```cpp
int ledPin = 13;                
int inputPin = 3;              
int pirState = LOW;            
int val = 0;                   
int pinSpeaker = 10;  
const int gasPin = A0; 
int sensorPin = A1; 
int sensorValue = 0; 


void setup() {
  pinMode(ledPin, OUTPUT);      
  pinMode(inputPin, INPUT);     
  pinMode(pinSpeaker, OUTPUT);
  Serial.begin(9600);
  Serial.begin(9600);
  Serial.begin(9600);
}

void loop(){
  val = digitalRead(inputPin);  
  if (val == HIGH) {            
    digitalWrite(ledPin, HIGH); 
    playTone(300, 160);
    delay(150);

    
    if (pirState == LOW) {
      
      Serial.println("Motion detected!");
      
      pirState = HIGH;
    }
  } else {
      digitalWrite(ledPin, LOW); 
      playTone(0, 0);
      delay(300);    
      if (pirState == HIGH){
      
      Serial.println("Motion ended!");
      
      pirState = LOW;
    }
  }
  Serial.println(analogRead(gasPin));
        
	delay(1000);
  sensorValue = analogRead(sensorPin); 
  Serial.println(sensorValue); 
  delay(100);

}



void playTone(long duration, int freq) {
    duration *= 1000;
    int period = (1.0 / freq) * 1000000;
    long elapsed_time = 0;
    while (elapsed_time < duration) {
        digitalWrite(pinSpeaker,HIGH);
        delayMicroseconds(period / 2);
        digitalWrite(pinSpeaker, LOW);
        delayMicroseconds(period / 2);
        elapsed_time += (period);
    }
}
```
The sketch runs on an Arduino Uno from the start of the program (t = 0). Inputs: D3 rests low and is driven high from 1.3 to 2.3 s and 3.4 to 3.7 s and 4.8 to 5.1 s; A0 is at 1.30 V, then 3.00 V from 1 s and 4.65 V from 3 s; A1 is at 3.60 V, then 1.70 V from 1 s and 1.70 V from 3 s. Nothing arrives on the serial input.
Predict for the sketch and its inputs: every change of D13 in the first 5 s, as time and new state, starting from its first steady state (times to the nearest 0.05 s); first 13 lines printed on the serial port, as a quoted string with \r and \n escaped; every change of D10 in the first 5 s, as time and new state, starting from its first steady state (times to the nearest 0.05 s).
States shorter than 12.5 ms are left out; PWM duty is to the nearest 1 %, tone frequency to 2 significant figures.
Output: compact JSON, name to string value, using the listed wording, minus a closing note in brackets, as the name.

{"every change of D13 in the first 5 s, as time and new state, starting from its first steady state": "0 s low; 1.4 s high; 2.95 s low", "first 13 lines printed on the serial port, as a quoted string with \\r and \\n escaped": "\"266\\r\\n348\\r\\nMotion detected!\\r\\n614\\r\\n348\\r\\nMotion ended!\\r\\n952\\r\\n348\\r\\n952\\r\\n348\\r\\n952\\r\\n348\\r\\n952\\r\\n\"", "every change of D10 in the first 5 s, as time and new state, starting from its first steady state": "0 s low; 1.4 s tone 160 Hz; 1.7 s low"}
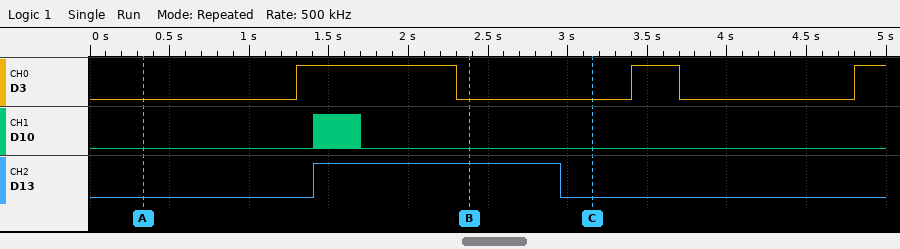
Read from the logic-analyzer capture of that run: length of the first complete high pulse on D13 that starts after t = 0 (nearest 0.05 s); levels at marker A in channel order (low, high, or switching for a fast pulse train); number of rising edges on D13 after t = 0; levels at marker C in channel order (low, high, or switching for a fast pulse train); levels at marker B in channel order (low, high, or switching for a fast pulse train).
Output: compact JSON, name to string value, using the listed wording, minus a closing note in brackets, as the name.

{"length of the first complete high pulse on D13 that starts after t = 0": "1.55 s", "levels at marker A in channel order": "D3 low, D10 low, D13 low", "number of rising edges on D13 after t = 0": "1", "levels at marker C in channel order": "D3 low, D10 low, D13 low", "levels at marker B in channel order": "D3 low, D10 low, D13 high"}
